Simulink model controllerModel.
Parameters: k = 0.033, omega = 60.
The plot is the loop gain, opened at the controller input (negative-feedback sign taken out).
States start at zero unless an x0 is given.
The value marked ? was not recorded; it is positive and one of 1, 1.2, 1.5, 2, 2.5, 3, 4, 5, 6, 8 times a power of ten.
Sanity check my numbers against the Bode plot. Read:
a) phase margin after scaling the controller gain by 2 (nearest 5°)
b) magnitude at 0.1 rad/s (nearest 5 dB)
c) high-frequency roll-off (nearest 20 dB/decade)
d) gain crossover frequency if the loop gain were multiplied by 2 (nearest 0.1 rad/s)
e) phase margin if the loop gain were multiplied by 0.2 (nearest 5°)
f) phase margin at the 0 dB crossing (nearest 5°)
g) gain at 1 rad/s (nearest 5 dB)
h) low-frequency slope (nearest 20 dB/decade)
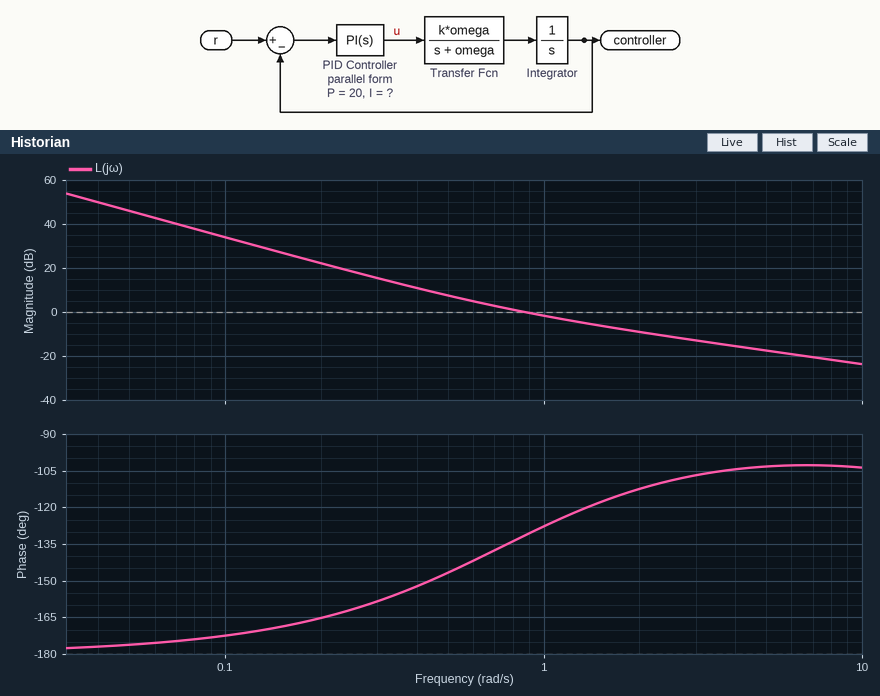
60°
35 dB
-20 dB/decade
1.5 rad/s
25°
50°
0 dB
-40 dB/decade
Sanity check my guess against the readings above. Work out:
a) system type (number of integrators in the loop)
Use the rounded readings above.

2
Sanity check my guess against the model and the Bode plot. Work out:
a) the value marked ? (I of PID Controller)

15
